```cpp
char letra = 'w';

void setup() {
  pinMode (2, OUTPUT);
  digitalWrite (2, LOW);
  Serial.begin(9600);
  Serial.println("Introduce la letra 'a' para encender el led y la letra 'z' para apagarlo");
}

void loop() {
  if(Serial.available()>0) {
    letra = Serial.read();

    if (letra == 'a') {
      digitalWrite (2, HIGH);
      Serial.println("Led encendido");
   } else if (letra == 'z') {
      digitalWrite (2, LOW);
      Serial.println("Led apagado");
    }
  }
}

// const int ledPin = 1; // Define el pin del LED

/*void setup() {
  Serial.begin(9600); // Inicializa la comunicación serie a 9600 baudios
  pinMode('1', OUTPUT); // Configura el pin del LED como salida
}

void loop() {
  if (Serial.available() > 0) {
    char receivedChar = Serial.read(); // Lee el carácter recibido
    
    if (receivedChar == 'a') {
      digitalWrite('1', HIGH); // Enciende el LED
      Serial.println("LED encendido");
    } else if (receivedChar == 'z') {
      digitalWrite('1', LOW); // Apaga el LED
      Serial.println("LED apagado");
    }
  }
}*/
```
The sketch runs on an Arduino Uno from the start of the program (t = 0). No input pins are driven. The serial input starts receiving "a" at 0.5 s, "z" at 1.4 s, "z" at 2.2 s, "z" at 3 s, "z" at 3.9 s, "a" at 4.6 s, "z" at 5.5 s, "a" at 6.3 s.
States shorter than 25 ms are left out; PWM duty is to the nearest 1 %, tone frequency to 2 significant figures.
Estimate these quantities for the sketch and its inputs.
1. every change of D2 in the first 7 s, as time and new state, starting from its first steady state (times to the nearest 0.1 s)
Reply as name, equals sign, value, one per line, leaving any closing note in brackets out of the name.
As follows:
every change of D2 in the first 7 s, as time and new state, starting from its first steady state = 0 s low; 0.5 s high; 1.4 s low; 4.6 s high; 5.5 s low; 6.3 s high
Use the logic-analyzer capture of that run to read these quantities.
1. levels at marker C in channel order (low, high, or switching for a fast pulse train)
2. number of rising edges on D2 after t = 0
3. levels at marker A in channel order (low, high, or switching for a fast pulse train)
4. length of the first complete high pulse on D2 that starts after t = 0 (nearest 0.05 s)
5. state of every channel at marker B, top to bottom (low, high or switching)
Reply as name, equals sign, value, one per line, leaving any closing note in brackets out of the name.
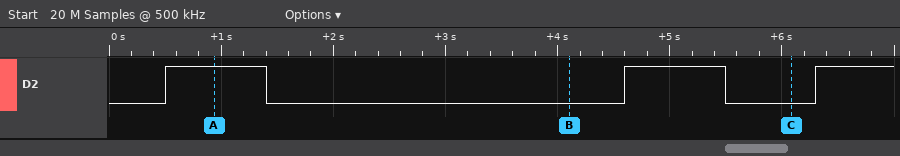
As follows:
levels at marker C in channel order = D2 low
number of rising edges on D2 after t = 0 = 3
levels at marker A in channel order = D2 high
length of the first complete high pulse on D2 that starts after t = 0 = 0.90 s
state of every channel at marker B, top to bottom = D2 low
